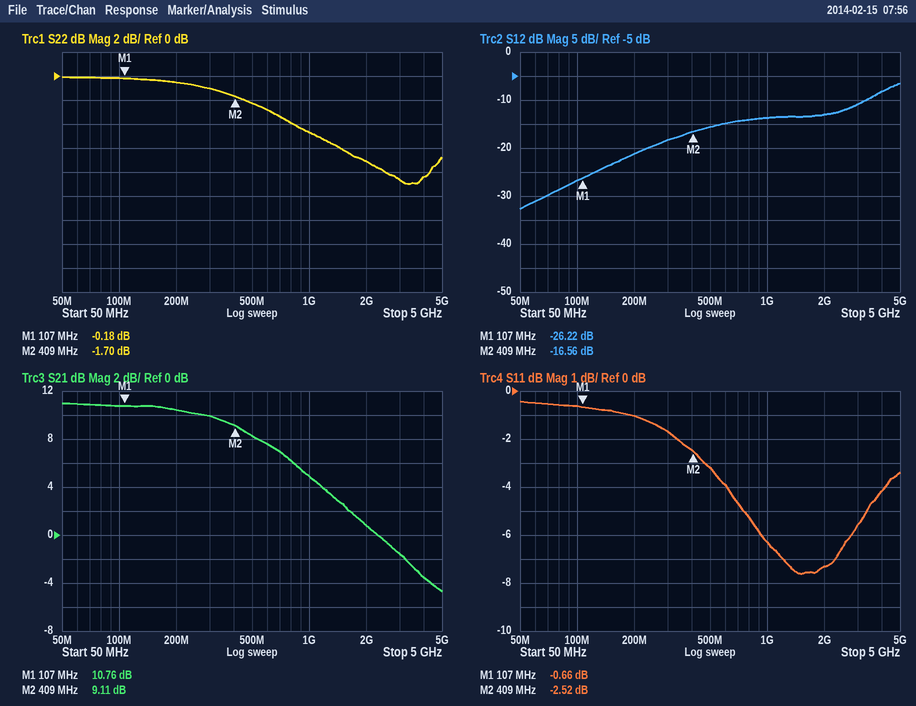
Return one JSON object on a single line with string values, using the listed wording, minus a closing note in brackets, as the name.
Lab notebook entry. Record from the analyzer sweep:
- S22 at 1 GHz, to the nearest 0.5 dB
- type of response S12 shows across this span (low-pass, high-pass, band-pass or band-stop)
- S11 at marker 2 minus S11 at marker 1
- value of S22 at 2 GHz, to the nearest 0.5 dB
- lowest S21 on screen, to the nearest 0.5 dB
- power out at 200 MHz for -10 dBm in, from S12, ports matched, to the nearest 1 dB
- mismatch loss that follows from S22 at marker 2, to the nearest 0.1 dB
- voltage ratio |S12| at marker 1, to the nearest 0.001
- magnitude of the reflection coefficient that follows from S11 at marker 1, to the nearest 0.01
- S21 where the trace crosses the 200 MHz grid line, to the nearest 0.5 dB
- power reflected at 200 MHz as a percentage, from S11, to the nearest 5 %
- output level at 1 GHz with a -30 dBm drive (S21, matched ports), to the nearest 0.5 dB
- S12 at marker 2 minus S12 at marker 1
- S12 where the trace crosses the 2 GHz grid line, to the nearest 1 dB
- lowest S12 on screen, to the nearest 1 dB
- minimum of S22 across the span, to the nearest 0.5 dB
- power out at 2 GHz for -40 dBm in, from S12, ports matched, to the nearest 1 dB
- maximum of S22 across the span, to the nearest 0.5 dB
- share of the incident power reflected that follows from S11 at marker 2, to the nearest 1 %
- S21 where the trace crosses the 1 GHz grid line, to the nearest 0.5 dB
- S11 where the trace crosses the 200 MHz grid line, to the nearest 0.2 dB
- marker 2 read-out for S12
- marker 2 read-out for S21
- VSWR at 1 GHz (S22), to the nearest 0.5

{"S22 at 1 GHz, to the nearest 0.5 dB": "-4.5 dB", "type of response S12 shows across this span": "high-pass", "S11 at marker 2 minus S11 at marker 1": "-1.86 dB", "value of S22 at 2 GHz, to the nearest 0.5 dB": "-7.0 dB", "lowest S21 on screen, to the nearest 0.5 dB": "-4.5 dB", "power out at 200 MHz for -10 dBm in, from S12, ports matched, to the nearest 1 dB": "-31 dBm", "mismatch loss that follows from S22 at marker 2, to the nearest 0.1 dB": "4.9 dB", "voltage ratio |S12| at marker 1, to the nearest 0.001": "0.049", "magnitude of the reflection coefficient that follows from S11 at marker 1, to the nearest 0.01": "0.93", "S21 where the trace crosses the 200 MHz grid line, to the nearest 0.5 dB": "10.5 dB", "power reflected at 200 MHz as a percentage, from S11, to the nearest 5 %": "80 %", "output level at 1 GHz with a -30 dBm drive (S21, matched ports), to the nearest 0.5 dB": "-25.0 dBm", "S12 at marker 2 minus S12 at marker 1": "9.66 dB", "S12 where the trace crosses the 2 GHz grid line, to the nearest 1 dB": "-13 dB", "lowest S12 on screen, to the nearest 1 dB": "-33 dB", "minimum of S22 across the span, to the nearest 0.5 dB": "-9.0 dB", "power out at 2 GHz for -40 dBm in, from S12, ports matched, to the nearest 1 dB": "-53 dBm", "maximum of S22 across the span, to the nearest 0.5 dB": "0.0 dB", "share of the incident power reflected that follows from S11 at marker 2, to the nearest 1 %": "56 %", "S21 where the trace crosses the 1 GHz grid line, to the nearest 0.5 dB": "5.0 dB", "S11 where the trace crosses the 200 MHz grid line, to the nearest 0.2 dB": "-1.0 dB", "marker 2 read-out for S12": "-16.56 dB", "marker 2 read-out for S21": "9.11 dB", "VSWR at 1 GHz (S22), to the nearest 0.5": "4.0"}
